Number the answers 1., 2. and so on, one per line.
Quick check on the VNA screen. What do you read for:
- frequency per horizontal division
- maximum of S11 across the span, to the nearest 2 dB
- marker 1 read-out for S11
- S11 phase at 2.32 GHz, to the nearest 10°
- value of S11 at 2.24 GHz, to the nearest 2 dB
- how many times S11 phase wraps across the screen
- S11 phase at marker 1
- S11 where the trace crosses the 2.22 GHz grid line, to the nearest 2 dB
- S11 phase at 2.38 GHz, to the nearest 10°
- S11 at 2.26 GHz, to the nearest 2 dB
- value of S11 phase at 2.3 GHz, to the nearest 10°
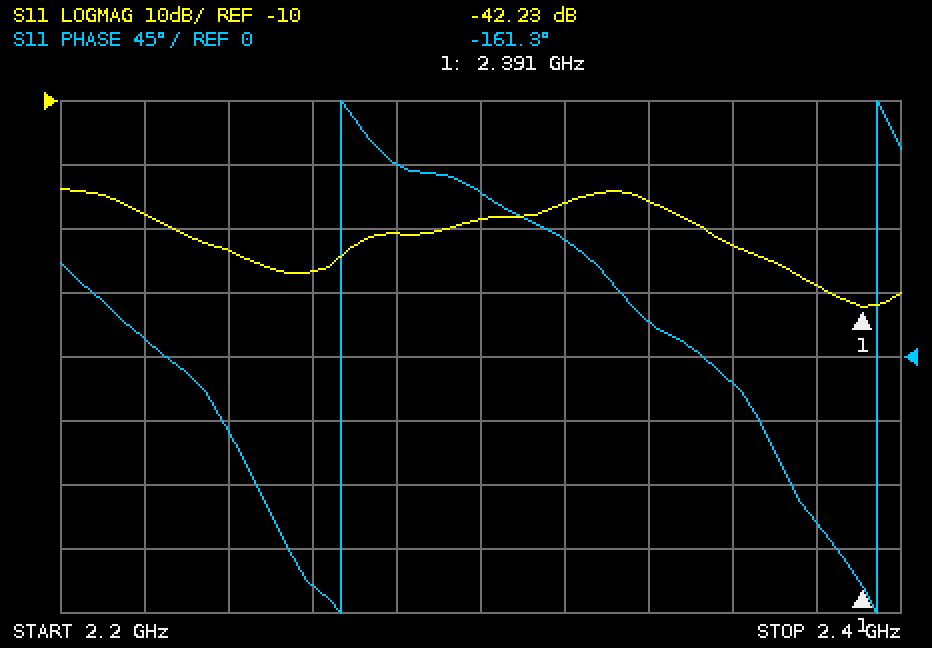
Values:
1. 20 MHz
2. -24 dB
3. -42.23 dB
4. 80°
5. -34 dB
6. 2
7. -161.3°
8. -28 dB
9. -120°
10. -36 dB
11. 120°
